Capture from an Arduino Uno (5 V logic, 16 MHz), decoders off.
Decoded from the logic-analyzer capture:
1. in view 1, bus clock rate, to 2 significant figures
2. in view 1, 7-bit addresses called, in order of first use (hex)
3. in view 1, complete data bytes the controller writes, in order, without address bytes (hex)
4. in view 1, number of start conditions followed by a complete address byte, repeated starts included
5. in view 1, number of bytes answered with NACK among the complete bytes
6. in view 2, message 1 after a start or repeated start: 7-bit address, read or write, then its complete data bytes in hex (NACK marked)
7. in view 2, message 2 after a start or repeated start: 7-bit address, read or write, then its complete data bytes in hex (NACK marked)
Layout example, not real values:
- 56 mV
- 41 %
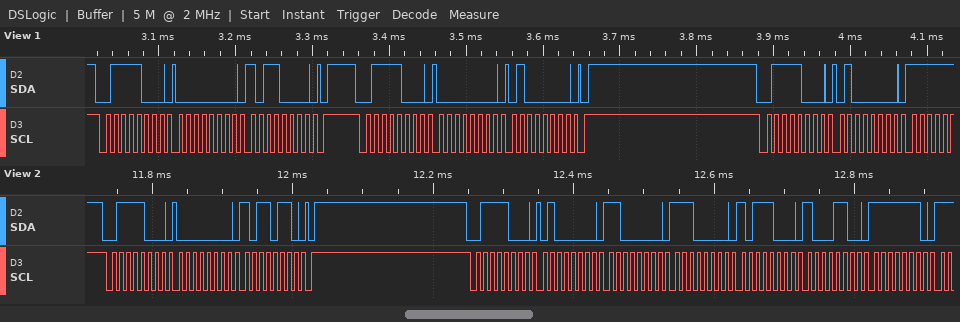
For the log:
- 100 kHz
- 0x3C
- 00 B0 00 40 40
- 3
- 0
- 0x3C write: 00 B6
- 0x3C write: 40 C0 E0 B8 8C FE
